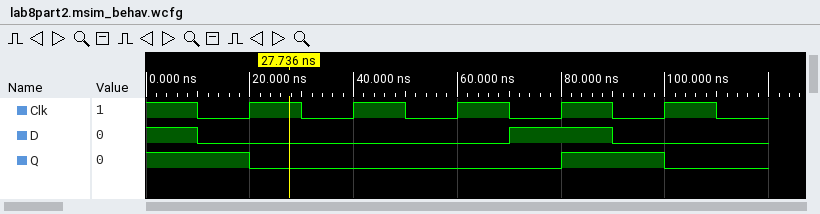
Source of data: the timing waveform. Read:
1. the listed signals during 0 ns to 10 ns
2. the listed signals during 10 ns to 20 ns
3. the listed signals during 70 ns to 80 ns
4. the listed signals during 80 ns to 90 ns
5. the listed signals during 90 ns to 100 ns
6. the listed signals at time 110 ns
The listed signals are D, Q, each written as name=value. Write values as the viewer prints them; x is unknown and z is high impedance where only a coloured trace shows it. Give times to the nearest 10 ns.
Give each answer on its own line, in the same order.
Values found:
D=1, Q=1
D=0, Q=1
D=1, Q=0
D=1, Q=1
D=0, Q=1
D=0, Q=0
